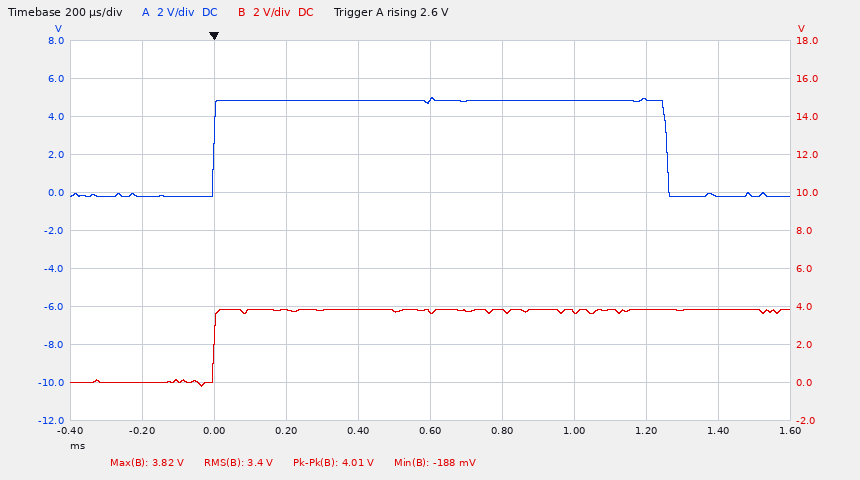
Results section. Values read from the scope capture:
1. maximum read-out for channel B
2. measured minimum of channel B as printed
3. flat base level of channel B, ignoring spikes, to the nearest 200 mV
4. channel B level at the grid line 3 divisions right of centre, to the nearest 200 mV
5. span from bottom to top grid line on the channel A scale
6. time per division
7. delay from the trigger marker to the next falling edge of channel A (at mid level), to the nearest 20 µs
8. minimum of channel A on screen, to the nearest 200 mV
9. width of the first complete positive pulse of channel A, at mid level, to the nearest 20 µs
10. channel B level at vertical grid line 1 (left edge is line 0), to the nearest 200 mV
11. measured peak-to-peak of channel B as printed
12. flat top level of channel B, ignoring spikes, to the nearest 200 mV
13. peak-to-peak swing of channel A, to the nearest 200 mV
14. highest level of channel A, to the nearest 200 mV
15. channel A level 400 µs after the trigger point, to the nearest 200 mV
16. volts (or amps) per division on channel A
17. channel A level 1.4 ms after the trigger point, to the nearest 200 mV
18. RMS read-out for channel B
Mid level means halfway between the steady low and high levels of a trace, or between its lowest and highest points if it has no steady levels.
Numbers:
3.82 V
-188 mV
0.0 V
3.8 V
20 V
200 µs
1.26 ms
-200 mV
1.26 ms
0.0 V
4.01 V
3.8 V
5.2 V
5.0 V
4.8 V
2 V
-200 mV
3.4 V
